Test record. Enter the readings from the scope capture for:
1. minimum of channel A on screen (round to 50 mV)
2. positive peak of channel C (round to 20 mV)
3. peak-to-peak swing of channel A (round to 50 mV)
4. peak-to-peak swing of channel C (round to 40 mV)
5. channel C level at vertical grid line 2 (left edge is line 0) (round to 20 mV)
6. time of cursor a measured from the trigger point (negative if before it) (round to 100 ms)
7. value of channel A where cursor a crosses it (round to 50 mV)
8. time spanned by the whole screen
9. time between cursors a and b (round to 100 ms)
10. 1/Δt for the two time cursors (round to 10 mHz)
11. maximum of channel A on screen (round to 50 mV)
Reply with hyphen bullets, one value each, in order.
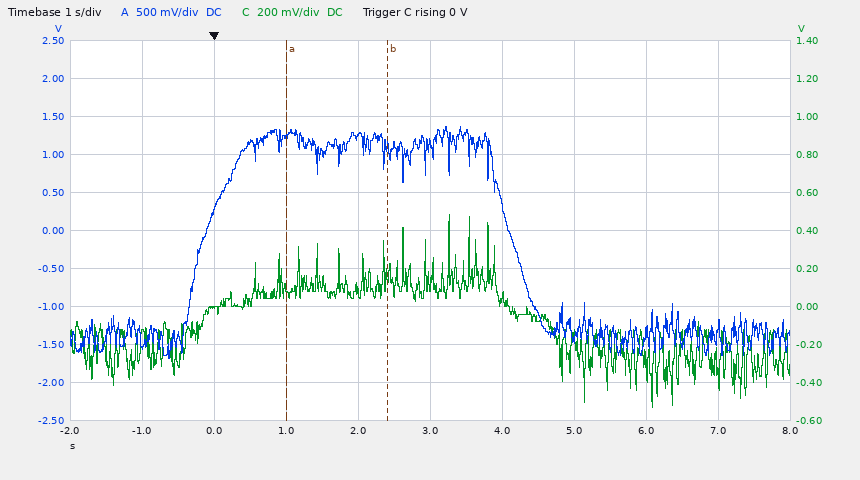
- -1.70 V
- 480 mV
- 3.05 V
- 1.00 V
- 0 mV
- +1.0 s
- 1.25 V
- 10 s
- 1.4 s
- 710 mHz
- 1.35 V
